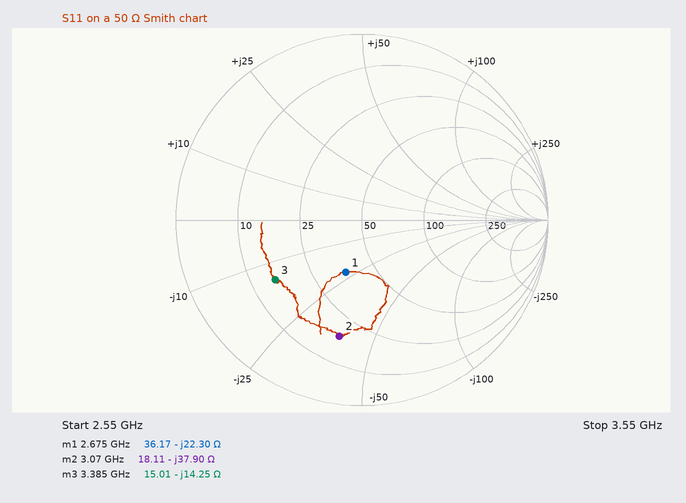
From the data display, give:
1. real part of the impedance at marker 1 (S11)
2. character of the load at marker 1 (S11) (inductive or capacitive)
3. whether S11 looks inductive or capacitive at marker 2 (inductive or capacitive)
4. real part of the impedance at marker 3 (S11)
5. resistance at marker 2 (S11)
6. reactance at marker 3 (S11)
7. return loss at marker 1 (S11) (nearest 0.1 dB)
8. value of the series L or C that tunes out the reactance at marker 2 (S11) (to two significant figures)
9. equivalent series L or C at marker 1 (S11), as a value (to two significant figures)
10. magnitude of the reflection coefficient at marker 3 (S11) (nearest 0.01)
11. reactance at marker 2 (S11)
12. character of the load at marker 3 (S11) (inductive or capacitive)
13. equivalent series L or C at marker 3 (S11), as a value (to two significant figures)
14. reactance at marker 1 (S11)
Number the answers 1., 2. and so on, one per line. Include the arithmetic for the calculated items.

1. 36.17 Ω
2. capacitive
3. capacitive
4. 15.01 Ω
5. 18.11 Ω
6. -14.25 Ω
7. 10.6 dB
8. L = 37.9 Ω/(2π × 3.07 GHz) ≈ 2.0 nH
9. C = 1/(2π × 2.675 GHz × 22.3 Ω) ≈ 2.7 pF
10. 0.57
11. -37.90 Ω
12. capacitive
13. C = 1/(2π × 3.385 GHz × 14.25 Ω) ≈ 3.3 pF
14. -22.30 Ω
